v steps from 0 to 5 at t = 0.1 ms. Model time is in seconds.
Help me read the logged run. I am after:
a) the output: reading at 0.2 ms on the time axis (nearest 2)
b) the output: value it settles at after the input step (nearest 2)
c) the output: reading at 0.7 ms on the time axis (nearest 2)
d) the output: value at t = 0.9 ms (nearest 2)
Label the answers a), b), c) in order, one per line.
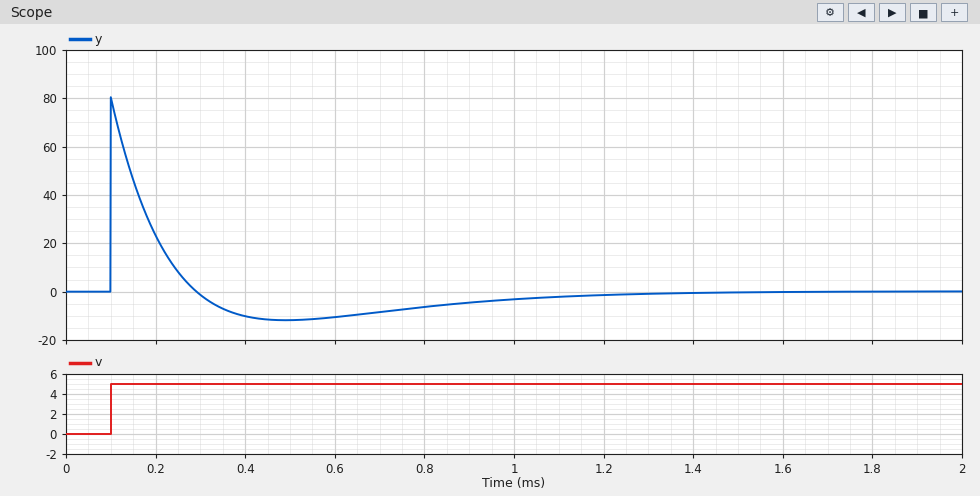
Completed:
a) 24
b) 0
c) -8
d) -4
